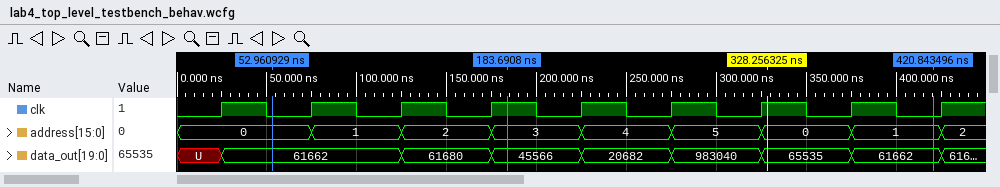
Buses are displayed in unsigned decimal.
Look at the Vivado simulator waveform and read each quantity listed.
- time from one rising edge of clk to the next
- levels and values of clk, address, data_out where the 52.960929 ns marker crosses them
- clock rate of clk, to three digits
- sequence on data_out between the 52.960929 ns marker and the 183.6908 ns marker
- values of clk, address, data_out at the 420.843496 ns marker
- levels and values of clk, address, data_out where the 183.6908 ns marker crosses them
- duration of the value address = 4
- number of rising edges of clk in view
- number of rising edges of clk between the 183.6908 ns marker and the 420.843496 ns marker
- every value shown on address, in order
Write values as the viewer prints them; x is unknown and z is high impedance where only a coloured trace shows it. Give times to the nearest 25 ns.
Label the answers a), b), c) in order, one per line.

a) 50 ns
b) clk=0, address=0, data_out=61662
c) 20.0 MHz
d) 61662, 61680, 45566
e) clk=0, address=1, data_out=61662
f) clk=1, address=3, data_out=45566
g) 50 ns
h) 9
i) 4
j) 0, 1, 2, 3, 4, 5, 0, 1, 2
